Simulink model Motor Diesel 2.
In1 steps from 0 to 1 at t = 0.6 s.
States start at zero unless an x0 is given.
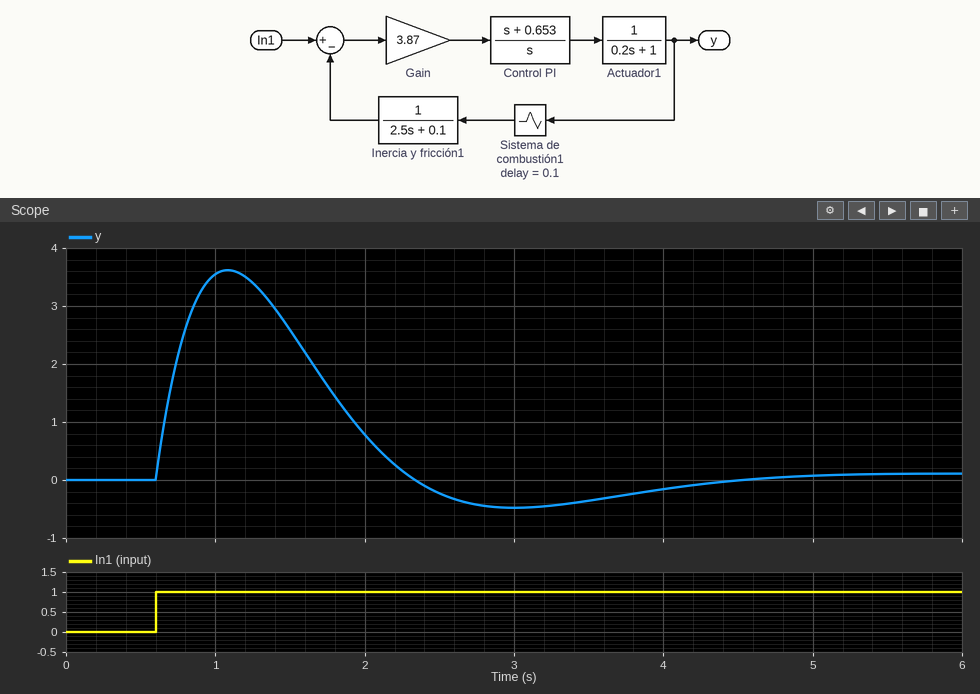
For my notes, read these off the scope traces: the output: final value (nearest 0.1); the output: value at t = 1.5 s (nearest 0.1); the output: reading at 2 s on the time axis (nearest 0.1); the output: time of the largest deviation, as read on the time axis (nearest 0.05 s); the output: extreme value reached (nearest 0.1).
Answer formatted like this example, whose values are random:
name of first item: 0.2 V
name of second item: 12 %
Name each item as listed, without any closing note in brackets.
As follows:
the output: final value: 0.1
the output: value at t = 1.5 s: 2.6
the output: reading at 2 s on the time axis: 0.8
the output: time of the largest deviation, as read on the time axis: 1.10 s
the output: extreme value reached: 3.6
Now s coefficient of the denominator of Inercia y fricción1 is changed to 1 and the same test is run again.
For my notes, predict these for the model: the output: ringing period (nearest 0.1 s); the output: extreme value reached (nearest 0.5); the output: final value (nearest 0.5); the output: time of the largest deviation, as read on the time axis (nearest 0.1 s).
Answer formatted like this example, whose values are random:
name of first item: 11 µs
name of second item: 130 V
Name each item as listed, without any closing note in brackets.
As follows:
the output: ringing period: 1.7 s
the output: extreme value reached: 3.0
the output: final value: 0.0
the output: time of the largest deviation, as read on the time axis: 0.9 s
